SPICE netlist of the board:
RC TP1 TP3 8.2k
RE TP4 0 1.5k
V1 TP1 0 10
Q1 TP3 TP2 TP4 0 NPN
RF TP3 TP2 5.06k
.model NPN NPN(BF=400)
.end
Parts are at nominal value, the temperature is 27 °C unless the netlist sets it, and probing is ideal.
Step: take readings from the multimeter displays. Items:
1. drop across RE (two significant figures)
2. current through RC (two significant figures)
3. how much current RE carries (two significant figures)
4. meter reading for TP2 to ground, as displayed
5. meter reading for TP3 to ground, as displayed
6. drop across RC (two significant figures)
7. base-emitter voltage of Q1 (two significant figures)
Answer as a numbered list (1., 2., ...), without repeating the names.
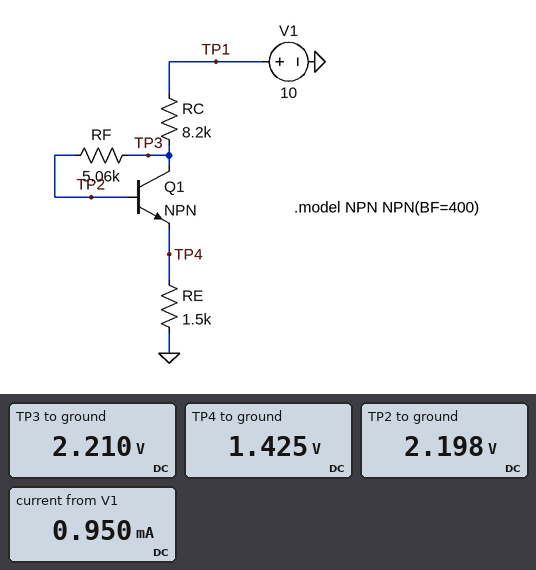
1. 1.4 V
2. 950 µA
3. 950 µA
4. 2.198 V
5. 2.210 V
6. 7.8 V
7. 770 mV
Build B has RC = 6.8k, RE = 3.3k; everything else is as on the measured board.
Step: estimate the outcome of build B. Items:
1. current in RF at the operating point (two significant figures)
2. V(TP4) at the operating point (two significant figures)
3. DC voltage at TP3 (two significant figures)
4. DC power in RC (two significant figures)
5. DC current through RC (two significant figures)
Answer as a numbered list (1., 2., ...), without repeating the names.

1. 2.3 µA
2. 3.0 V
3. 3.8 V
4. 5.7 mW
5. 910 µA
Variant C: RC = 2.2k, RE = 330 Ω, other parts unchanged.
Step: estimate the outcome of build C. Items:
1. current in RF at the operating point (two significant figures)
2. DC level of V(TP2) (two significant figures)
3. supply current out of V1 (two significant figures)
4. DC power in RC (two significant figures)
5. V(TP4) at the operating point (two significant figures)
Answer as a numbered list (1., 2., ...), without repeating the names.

1. 9.0 µA
2. 2.0 V
3. 3.6 mA
4. 29 mW
5. 1.2 V
